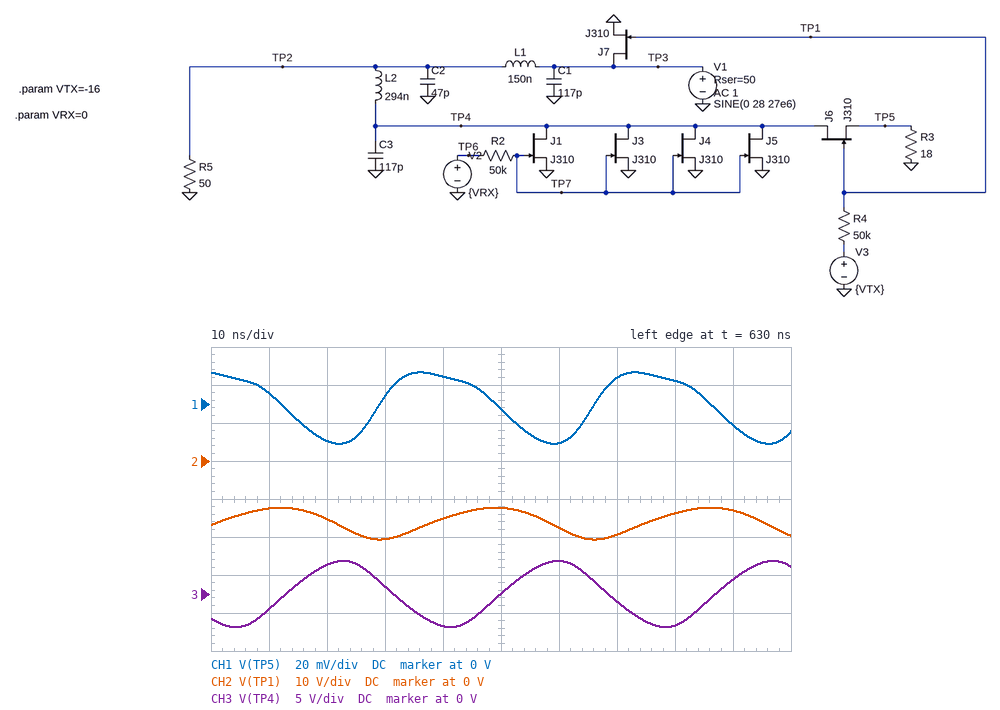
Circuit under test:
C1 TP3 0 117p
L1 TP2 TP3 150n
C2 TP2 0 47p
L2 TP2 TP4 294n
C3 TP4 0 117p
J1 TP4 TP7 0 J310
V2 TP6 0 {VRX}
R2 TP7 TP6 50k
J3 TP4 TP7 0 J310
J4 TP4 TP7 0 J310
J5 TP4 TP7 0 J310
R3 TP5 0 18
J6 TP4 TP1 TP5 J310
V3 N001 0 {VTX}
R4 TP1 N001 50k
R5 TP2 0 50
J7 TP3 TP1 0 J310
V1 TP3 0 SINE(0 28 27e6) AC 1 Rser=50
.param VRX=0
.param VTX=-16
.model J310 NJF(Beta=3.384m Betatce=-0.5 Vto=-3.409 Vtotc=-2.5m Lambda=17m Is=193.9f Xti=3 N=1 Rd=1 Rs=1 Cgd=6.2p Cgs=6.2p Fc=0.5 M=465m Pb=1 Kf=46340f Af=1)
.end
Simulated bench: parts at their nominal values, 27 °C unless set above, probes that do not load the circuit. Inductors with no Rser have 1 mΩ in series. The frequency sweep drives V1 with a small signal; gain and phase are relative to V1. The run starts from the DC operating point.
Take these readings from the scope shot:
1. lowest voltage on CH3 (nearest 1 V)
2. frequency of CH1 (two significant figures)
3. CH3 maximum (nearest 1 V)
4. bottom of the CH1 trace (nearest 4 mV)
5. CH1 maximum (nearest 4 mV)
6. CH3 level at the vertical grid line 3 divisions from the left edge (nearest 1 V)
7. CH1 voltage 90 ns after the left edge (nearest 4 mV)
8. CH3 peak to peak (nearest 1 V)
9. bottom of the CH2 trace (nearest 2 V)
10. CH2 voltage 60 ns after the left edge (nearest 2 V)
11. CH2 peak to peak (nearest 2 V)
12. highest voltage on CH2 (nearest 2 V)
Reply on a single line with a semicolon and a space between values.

-4 V; 27 MHz; 4 V; -20 mV; 16 mV; 1 V; -12 mV; 9 V; -20 V; -18 V; 8 V; -12 V
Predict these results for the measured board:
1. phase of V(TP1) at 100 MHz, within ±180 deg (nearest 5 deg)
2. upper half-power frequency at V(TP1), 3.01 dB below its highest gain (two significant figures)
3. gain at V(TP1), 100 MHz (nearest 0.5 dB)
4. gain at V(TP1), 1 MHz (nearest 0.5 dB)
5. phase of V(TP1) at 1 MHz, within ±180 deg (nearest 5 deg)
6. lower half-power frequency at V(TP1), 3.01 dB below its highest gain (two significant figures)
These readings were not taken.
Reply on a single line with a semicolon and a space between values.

-65 deg; 54 MHz; -22.5 dB; -23.0 dB; 30 deg; 8.8 MHz
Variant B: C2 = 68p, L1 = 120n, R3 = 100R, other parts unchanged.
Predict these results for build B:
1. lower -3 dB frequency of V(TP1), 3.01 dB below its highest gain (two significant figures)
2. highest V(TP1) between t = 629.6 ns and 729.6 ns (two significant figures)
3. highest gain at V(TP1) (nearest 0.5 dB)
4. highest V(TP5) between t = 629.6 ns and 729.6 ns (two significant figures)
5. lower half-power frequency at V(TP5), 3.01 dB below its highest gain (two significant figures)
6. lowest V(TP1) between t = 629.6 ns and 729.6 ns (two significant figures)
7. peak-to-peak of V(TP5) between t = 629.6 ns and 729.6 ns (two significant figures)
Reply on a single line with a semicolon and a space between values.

7.7 MHz; -13 V; -17.5 dB; 77 mV; 64 MHz; -20 V; 180 mV
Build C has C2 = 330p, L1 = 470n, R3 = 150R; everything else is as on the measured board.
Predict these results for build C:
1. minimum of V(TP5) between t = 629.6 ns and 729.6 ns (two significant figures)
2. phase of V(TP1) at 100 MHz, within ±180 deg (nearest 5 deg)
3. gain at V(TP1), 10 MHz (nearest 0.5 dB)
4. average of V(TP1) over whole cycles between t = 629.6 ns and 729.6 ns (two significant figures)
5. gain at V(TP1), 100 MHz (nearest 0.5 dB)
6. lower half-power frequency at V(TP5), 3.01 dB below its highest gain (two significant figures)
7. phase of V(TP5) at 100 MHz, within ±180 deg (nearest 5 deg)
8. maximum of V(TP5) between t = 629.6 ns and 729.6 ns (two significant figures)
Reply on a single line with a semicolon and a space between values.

-230 mV; -70 deg; -17.0 dB; -16 V; -23.5 dB; 26 MHz; 10 deg; 240 mV
